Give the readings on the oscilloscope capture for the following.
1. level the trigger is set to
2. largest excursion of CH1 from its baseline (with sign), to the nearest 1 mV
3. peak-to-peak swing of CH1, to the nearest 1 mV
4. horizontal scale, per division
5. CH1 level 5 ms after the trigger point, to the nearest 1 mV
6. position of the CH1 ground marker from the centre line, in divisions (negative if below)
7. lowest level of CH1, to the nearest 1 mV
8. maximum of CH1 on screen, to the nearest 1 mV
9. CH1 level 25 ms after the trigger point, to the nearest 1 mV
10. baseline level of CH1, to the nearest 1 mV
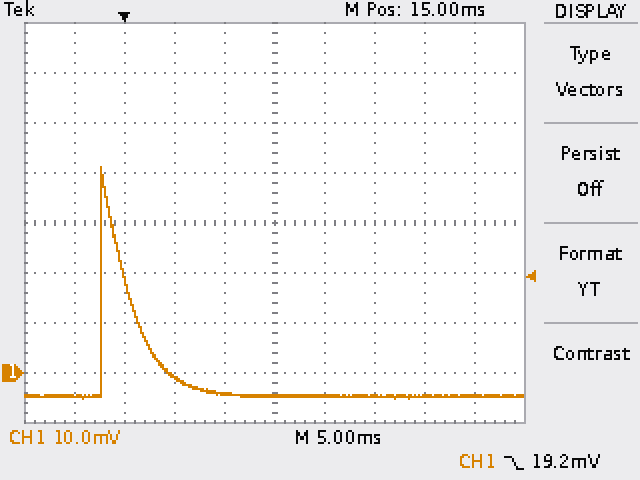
19.2 mV
+46 mV
46 mV
5 ms
-1 mV
-3.0 div
-5 mV
41 mV
-5 mV
-5 mV
